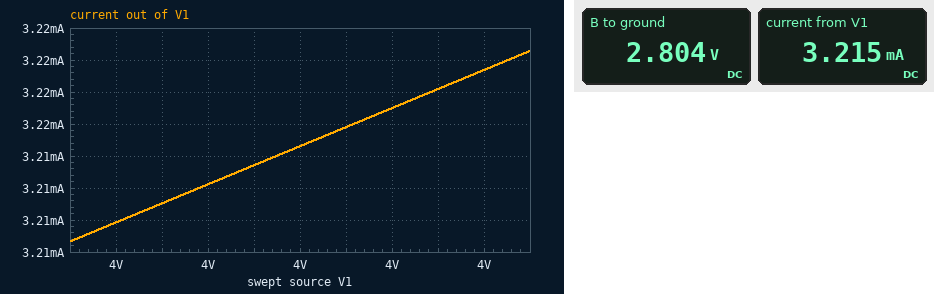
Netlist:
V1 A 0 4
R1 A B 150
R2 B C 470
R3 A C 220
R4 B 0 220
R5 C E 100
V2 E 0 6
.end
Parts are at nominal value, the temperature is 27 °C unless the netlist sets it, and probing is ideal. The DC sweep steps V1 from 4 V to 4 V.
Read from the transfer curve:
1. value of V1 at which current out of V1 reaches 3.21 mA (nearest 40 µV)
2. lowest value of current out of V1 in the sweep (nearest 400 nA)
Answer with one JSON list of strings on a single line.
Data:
["3.99956 V", "3.2088 mA"]
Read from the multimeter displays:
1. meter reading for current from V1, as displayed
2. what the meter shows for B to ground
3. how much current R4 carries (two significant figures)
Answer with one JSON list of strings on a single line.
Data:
["3.215 mA", "2.804 V", "13 mA"]
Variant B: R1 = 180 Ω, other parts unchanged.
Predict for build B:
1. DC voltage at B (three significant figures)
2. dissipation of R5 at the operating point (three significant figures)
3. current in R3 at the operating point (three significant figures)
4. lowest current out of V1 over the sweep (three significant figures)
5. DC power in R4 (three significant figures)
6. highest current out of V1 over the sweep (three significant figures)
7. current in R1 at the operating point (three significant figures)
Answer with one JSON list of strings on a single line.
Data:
["2.69 V", "9.36 mW", "4.69 mA", "2.56 mA", "33.0 mW", "2.57 mA", "7.26 mA"]
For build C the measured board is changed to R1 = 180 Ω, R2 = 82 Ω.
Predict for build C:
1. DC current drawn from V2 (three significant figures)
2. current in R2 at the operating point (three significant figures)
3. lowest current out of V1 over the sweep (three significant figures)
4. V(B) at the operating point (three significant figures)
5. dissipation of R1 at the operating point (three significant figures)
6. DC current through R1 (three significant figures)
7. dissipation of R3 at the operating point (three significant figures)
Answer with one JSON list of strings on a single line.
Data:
["15.0 mA", "12.7 mA", "725 µA", "3.46 V", "1.63 mW", "3.01 mA", "1.14 mW"]
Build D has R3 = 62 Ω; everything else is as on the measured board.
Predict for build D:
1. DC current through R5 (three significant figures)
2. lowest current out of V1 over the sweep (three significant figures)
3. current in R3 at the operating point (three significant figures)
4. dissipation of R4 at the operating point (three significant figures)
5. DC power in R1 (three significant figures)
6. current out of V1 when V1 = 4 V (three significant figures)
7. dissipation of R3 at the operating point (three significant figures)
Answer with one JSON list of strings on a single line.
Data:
["13.9 mA", "-1.45 mA", "9.88 mA", "34.0 mW", "10.7 mW", "-1.44 mA", "6.05 mW"]
